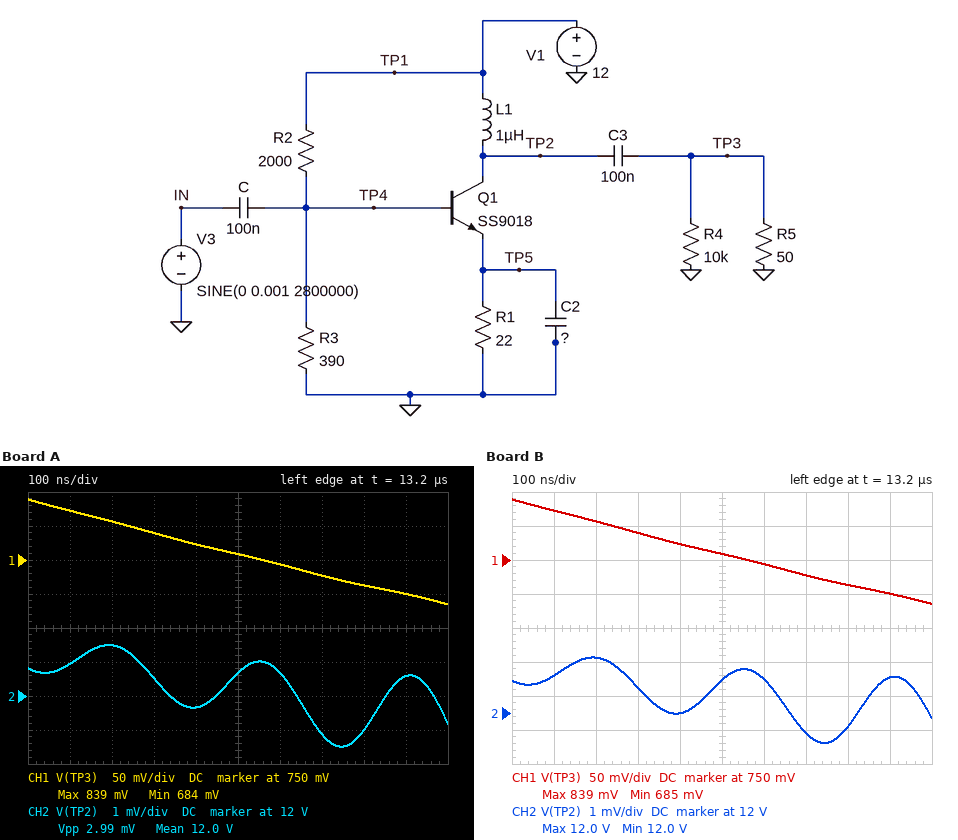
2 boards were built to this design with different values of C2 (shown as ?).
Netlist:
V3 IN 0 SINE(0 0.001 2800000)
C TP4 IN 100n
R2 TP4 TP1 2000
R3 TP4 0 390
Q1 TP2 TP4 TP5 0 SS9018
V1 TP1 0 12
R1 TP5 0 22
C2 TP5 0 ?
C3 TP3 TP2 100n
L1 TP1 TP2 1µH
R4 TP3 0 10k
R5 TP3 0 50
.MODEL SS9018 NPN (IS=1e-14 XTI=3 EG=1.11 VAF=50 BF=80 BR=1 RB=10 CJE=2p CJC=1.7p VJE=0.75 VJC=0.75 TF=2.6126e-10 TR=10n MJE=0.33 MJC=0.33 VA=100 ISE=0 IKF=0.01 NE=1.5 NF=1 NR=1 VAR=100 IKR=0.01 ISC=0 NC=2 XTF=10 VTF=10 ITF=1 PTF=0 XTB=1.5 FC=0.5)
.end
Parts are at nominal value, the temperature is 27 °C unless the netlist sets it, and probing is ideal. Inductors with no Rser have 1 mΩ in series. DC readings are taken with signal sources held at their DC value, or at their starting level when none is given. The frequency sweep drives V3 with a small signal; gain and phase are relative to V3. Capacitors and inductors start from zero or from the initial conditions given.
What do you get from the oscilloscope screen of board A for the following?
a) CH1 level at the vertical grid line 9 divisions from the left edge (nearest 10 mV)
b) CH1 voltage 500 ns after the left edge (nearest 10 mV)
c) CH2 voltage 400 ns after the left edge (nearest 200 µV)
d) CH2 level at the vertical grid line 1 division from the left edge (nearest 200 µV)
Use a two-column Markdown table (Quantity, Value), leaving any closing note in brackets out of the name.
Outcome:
| Quantity | Value |
|---|---|
| CH1 level at the vertical grid line 9 divisions from the left edge | 700 mV |
| CH1 voltage 500 ns after the left edge | 760 mV |
| CH2 voltage 400 ns after the left edge | 12.0006 V |
| CH2 level at the vertical grid line 1 division from the left edge | 12.0020 V |
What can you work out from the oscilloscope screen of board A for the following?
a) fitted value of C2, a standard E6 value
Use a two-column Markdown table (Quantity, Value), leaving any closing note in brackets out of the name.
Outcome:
| Quantity | Value |
|---|---|
| fitted value of C2, a standard E6 value | 330 nF |
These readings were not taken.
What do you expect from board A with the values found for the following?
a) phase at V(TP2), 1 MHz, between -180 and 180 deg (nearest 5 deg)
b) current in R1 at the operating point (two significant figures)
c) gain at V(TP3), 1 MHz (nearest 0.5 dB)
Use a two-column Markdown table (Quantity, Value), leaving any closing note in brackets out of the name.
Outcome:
| Quantity | Value |
|---|---|
| phase at V(TP2), 1 MHz, between -180 and 180 deg | -80 deg |
| current in R1 at the operating point | 33 mA |
| gain at V(TP3), 1 MHz | 8.5 dB |
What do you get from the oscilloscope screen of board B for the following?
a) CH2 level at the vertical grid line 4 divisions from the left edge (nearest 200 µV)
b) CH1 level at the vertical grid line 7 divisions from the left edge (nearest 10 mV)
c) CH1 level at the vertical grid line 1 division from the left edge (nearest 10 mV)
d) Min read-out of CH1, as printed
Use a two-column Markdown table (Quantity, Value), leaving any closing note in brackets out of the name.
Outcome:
| Quantity | Value |
|---|---|
| CH2 level at the vertical grid line 4 divisions from the left edge | 12.0010 V |
| CH1 level at the vertical grid line 7 divisions from the left edge | 730 mV |
| CH1 level at the vertical grid line 1 division from the left edge | 820 mV |
| Min read-out of CH1, as printed | 685 mV |
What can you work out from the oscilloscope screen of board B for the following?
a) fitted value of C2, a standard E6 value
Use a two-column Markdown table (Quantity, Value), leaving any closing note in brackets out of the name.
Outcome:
| Quantity | Value |
|---|---|
| fitted value of C2, a standard E6 value | 150 nF |
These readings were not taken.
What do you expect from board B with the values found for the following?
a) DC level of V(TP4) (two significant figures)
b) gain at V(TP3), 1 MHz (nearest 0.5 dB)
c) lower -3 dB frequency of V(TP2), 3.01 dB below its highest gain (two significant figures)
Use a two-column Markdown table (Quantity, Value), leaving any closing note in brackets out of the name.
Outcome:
| Quantity | Value |
|---|---|
| DC level of V(TP4) | 1.5 V |
| gain at V(TP3), 1 MHz | 7.5 dB |
| lower -3 dB frequency of V(TP2), 3.01 dB below its highest gain | 6.9 MHz |
